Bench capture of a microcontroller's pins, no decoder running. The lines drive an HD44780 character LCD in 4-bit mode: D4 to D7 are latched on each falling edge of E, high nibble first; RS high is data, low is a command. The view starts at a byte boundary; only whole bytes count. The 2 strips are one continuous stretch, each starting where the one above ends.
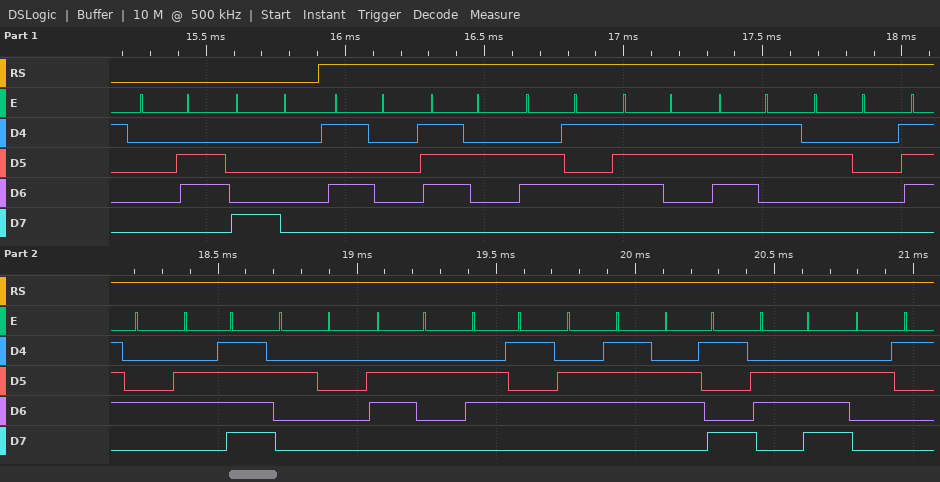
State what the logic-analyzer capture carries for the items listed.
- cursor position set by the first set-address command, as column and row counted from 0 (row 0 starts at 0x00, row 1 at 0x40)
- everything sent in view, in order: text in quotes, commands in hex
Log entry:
column 0, row 0
0x06 0x80 "Press to begin!"
